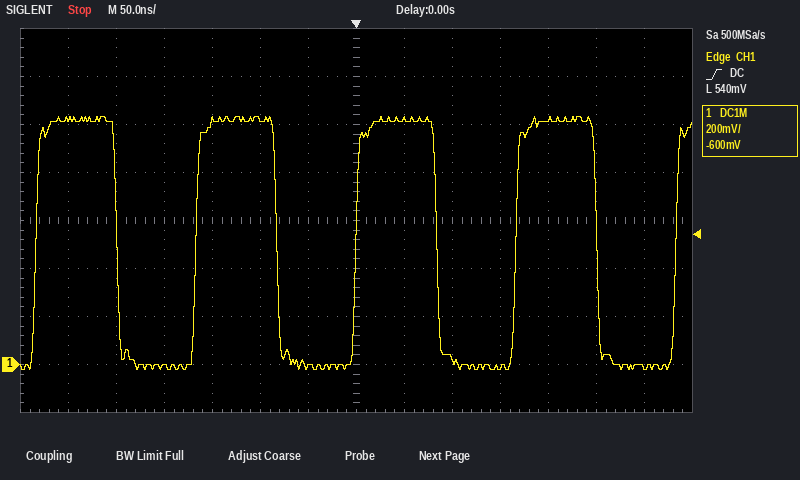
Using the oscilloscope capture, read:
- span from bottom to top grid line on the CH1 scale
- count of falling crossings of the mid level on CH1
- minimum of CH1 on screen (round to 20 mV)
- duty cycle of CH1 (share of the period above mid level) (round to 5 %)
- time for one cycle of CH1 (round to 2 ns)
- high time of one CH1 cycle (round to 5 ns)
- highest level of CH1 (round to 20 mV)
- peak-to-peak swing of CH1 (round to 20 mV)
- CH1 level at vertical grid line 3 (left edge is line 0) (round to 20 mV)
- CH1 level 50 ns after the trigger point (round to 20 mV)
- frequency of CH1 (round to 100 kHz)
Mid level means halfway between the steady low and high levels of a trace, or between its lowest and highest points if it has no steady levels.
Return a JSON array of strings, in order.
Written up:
["1.6 V", "4", "-20 mV", "50 %", "166 ns", "85 ns", "1.04 V", "1.06 V", "0 mV", "1.02 V", "6.0 MHz"]
